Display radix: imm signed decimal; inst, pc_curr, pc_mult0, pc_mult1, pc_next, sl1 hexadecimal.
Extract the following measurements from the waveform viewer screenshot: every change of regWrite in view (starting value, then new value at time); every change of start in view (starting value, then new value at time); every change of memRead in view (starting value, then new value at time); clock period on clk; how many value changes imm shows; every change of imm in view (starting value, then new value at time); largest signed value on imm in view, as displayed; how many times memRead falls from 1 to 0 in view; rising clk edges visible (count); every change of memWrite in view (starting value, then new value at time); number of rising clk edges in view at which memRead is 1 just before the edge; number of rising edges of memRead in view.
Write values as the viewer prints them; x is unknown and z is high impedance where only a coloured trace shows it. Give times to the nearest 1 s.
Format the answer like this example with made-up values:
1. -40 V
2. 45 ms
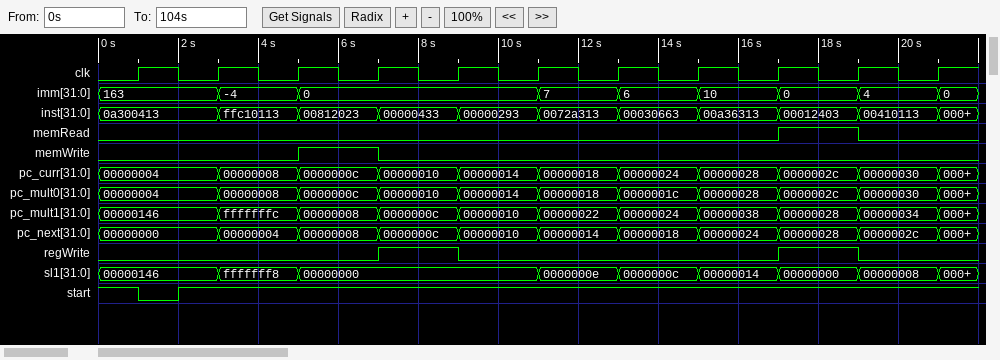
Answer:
1. 0, 1 at 7 s, 0 at 9 s, 1 at 17 s, 0 at 19 s
2. 1, 0 at 1 s, 1 at 2 s
3. 0, 1 at 17 s, 0 at 19 s
4. 2 s
5. 8
6. 163, -4 at 3 s, 0 at 5 s, 7 at 11 s, 6 at 13 s, 10 at 15 s, 0 at 17 s, 4 at 19 s, 0 at 21 s
7. 163
8. 1
9. 11
10. 0, 1 at 5 s, 0 at 7 s
11. 1
12. 1
